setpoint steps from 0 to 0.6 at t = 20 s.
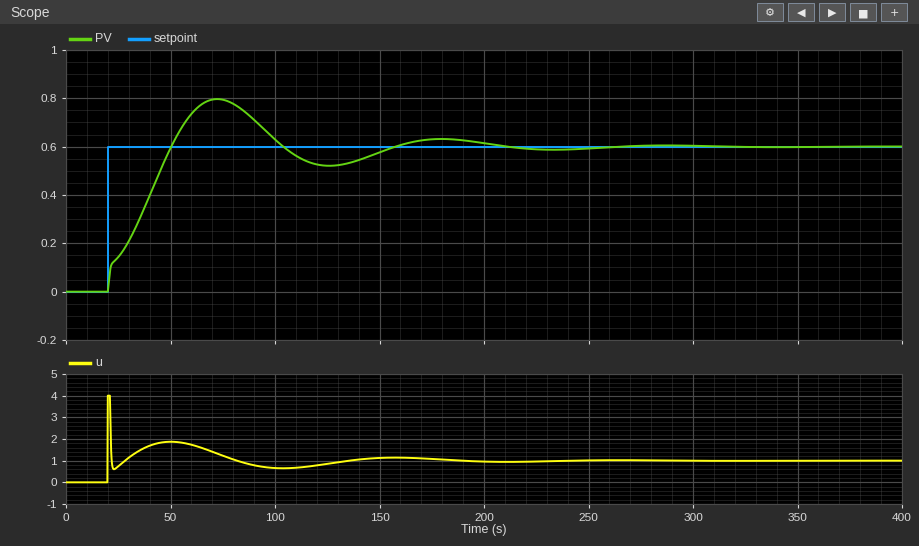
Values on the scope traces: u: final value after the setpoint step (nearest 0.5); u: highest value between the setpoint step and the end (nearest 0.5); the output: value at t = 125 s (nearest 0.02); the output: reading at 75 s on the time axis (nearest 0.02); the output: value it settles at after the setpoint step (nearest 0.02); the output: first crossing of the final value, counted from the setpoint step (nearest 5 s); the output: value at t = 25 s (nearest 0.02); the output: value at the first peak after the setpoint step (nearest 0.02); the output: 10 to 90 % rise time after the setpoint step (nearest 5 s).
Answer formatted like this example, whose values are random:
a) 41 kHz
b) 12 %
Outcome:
a) 1.0
b) 4.0
c) 0.52
d) 0.80
e) 0.60
f) 30 s
g) 0.14
h) 0.80
i) 25 s
